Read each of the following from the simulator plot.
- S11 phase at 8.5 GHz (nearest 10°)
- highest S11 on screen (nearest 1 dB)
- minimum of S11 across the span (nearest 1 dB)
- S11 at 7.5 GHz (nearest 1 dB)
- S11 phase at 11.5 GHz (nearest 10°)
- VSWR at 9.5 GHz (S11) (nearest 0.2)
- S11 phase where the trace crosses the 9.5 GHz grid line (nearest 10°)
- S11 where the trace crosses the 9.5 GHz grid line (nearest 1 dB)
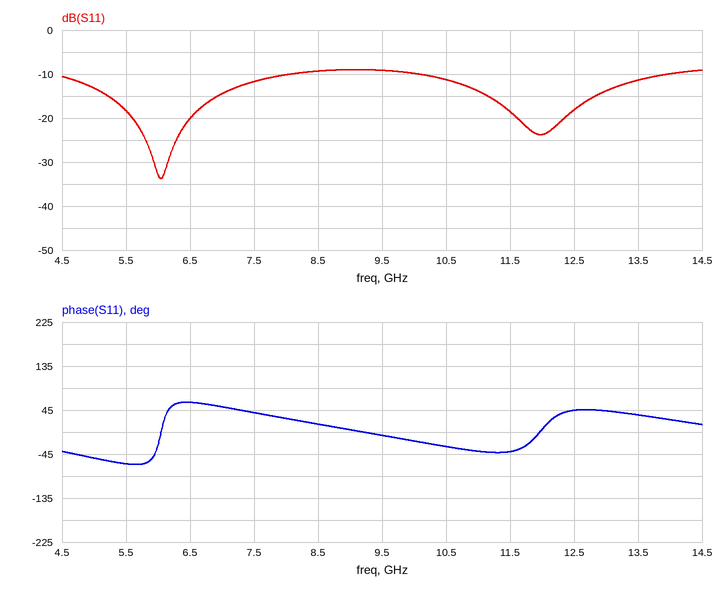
20°
-9 dB
-34 dB
-12 dB
-40°
2.0
-10°
-9 dB
